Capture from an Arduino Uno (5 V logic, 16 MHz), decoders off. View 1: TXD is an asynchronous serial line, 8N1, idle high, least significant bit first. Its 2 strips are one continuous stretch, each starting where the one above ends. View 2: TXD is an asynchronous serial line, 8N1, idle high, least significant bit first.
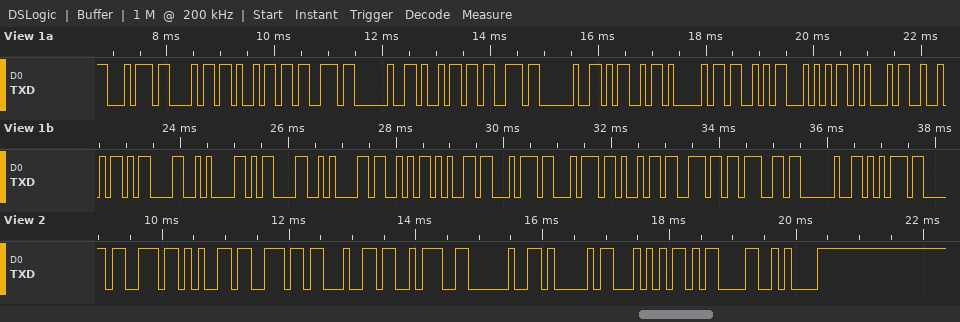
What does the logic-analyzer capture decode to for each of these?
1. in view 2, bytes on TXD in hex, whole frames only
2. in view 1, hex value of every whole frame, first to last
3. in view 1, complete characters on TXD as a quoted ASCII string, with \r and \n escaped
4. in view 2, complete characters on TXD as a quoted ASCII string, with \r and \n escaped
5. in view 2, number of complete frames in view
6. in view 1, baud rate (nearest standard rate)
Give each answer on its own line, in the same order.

0x73 0x65 0x6E 0x64 0x3A 0x20 0x41 0x54 0x0D 0x0A
74 68 69 73 20 69 73 20 4D 41 53 54 45 52 0D 0A 0D 0A 53 65 74 74 69 6E 67 20 75
"this is MASTER\r\n\r\nSetting u"
"send: AT\r\n"
10
9600 baud
